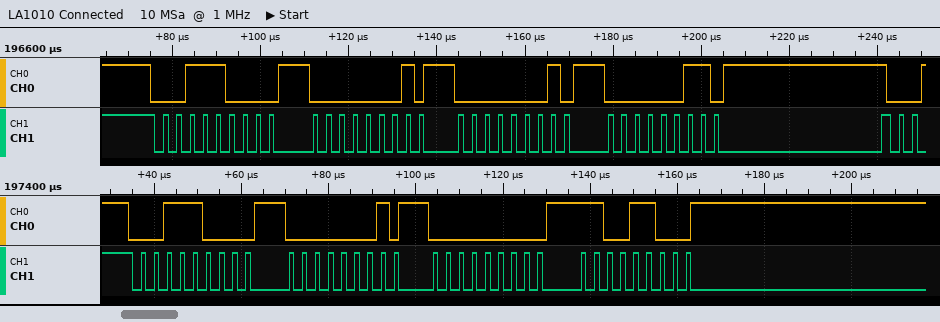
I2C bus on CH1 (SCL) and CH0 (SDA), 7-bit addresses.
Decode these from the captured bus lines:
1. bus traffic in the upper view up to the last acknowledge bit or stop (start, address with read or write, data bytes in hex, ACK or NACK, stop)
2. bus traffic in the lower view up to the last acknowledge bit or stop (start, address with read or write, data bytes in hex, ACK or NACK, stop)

start, address 1C write ACK, 01 ACK, 01 ACK, 03 ACK
start, address 1C write ACK, 01 ACK, 00 ACK, CC ACK
